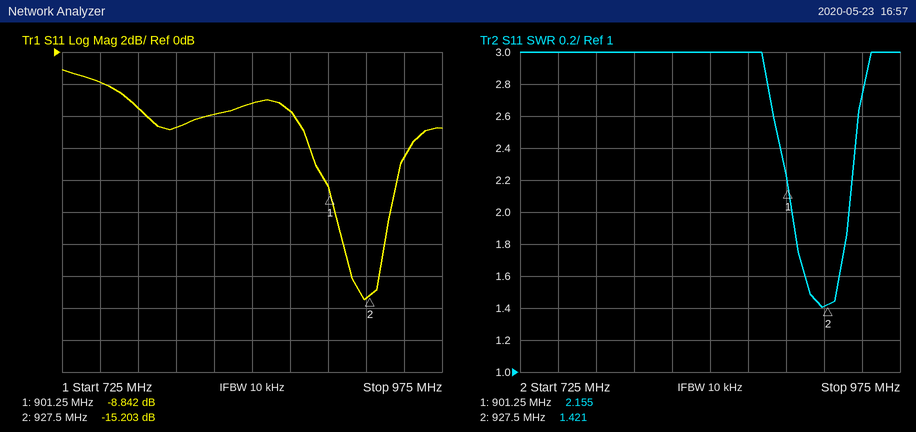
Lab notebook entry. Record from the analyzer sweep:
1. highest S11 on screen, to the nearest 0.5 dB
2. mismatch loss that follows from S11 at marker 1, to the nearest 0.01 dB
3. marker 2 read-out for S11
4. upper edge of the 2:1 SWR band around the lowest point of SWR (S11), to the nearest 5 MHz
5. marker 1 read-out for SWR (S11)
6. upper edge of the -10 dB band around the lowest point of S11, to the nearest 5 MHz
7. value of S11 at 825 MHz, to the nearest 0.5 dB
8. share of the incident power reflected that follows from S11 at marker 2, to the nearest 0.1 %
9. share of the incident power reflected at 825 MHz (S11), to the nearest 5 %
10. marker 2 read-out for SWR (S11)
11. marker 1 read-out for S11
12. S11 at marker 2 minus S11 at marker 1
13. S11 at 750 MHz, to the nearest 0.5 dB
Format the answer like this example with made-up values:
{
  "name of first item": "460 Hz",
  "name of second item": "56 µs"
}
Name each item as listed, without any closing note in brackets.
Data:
{
  "highest S11 on screen, to the nearest 0.5 dB": "-1.0 dB",
  "mismatch loss that follows from S11 at marker 1, to the nearest 0.01 dB": "0.61 dB",
  "marker 2 read-out for S11": "-15.203 dB",
  "upper edge of the 2:1 SWR band around the lowest point of SWR (S11), to the nearest 5 MHz": "940 MHz",
  "marker 1 read-out for SWR": "2.155",
  "upper edge of the -10 dB band around the lowest point of S11, to the nearest 5 MHz": "940 MHz",
  "value of S11 at 825 MHz, to the nearest 0.5 dB": "-4.0 dB",
  "share of the incident power reflected that follows from S11 at marker 2, to the nearest 0.1 %": "3.0 %",
  "share of the incident power reflected at 825 MHz (S11), to the nearest 5 %": "40 %",
  "marker 2 read-out for SWR": "1.421",
  "marker 1 read-out for S11": "-8.842 dB",
  "S11 at marker 2 minus S11 at marker 1": "-6.361 dB",
  "S11 at 750 MHz, to the nearest 0.5 dB": "-2.0 dB"
}
